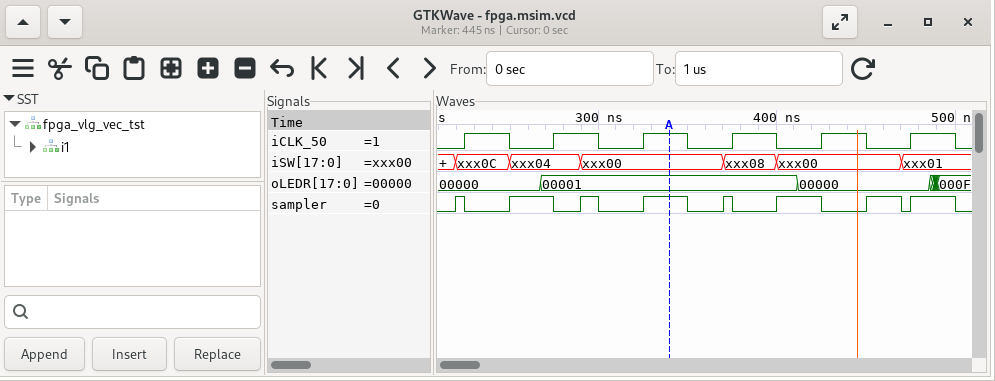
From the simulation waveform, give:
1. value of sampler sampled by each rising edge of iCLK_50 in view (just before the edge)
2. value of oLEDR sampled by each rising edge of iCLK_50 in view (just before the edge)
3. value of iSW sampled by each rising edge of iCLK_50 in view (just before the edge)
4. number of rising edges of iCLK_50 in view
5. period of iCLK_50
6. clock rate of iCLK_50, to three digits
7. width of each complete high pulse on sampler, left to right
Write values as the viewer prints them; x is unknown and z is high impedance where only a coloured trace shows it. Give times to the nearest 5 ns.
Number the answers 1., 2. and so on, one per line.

1. 1 1 0 1 1 0
2. 00000, 00001, 00001, 00001, 00000, 00000
3. xxx0C, xxx04, xxx00, xxx08, xxx00, xxx01
4. 6
5. 50 ns
6. 20.0 MHz
7. 5 ns, 25 ns, 10 ns, 25 ns, 5 ns, 25 ns, 20 ns, 25 ns
